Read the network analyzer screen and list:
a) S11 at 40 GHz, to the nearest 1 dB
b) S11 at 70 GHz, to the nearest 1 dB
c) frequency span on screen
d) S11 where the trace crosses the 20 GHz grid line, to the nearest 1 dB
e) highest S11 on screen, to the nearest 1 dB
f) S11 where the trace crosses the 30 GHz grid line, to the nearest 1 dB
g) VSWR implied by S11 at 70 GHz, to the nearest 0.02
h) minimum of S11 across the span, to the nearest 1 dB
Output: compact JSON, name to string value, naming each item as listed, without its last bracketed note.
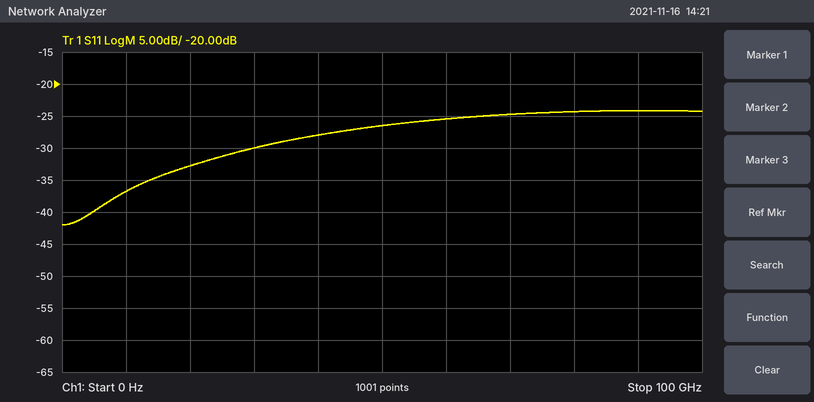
{"S11 at 40 GHz, to the nearest 1 dB": "-28 dB", "S11 at 70 GHz, to the nearest 1 dB": "-25 dB", "frequency span on screen": "100 GHz", "S11 where the trace crosses the 20 GHz grid line, to the nearest 1 dB": "-33 dB", "highest S11 on screen, to the nearest 1 dB": "-24 dB", "S11 where the trace crosses the 30 GHz grid line, to the nearest 1 dB": "-30 dB", "VSWR implied by S11 at 70 GHz, to the nearest 0.02": "1.12", "minimum of S11 across the span, to the nearest 1 dB": "-42 dB"}
